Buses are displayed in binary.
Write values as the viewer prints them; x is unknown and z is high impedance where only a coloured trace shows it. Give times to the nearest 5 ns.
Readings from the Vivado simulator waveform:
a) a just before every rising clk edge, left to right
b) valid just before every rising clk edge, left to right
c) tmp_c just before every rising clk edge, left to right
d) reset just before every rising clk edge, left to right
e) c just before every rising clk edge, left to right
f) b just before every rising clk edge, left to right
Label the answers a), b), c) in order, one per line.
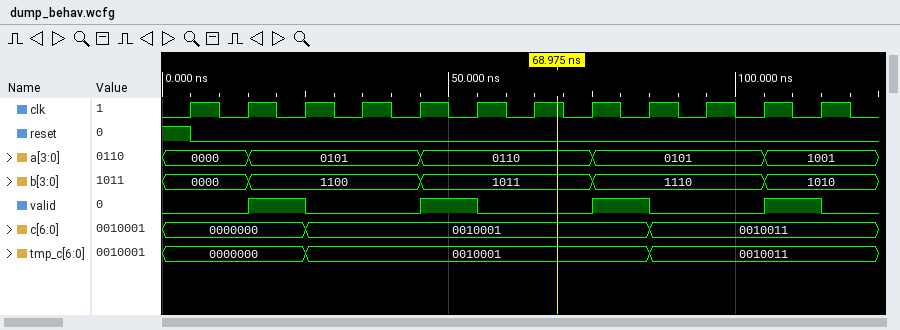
a) 0000, 0000, 0101, 0101, 0101, 0110, 0110, 0110, 0101, 0101, 0101, 1001
b) 0 0 1 0 0 1 0 0 1 0 0 1
c) 0000000, 0000000, 0000000, 0010001, 0010001, 0010001, 0010001, 0010001, 0010001, 0010011, 0010011, 0010011
d) 1 0 0 0 0 0 0 0 0 0 0 0
e) 0000000, 0000000, 0000000, 0010001, 0010001, 0010001, 0010001, 0010001, 0010001, 0010011, 0010011, 0010011
f) 0000, 0000, 1100, 1100, 1100, 1011, 1011, 1011, 1110, 1110, 1110, 1010
